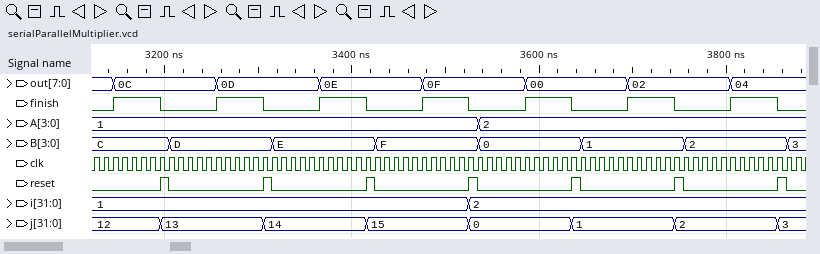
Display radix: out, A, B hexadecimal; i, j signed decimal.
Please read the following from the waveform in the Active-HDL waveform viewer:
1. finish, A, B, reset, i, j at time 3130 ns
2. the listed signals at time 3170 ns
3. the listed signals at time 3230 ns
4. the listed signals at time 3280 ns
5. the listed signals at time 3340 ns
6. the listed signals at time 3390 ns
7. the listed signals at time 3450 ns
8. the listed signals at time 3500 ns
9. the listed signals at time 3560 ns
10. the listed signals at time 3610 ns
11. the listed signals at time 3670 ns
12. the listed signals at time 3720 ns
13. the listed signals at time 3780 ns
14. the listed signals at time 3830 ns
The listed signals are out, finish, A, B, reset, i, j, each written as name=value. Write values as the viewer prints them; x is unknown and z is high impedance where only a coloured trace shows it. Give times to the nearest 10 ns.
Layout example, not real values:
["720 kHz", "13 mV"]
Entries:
["finish=0, A=1, B=C, reset=0, i=1, j=12", "out=0C, finish=1, A=1, B=C, reset=0, i=1, j=12", "out=0C, finish=0, A=1, B=D, reset=0, i=1, j=13", "out=0D, finish=1, A=1, B=D, reset=0, i=1, j=13", "out=0D, finish=0, A=1, B=E, reset=0, i=1, j=14", "out=0E, finish=1, A=1, B=E, reset=0, i=1, j=14", "out=0E, finish=0, A=1, B=F, reset=0, i=1, j=15", "out=0F, finish=1, A=1, B=F, reset=0, i=1, j=15", "out=0F, finish=0, A=2, B=0, reset=0, i=2, j=0", "out=00, finish=1, A=2, B=0, reset=0, i=2, j=0", "out=00, finish=0, A=2, B=1, reset=0, i=2, j=1", "out=02, finish=1, A=2, B=1, reset=0, i=2, j=1", "out=02, finish=0, A=2, B=2, reset=0, i=2, j=2", "out=04, finish=1, A=2, B=2, reset=0, i=2, j=2"]
